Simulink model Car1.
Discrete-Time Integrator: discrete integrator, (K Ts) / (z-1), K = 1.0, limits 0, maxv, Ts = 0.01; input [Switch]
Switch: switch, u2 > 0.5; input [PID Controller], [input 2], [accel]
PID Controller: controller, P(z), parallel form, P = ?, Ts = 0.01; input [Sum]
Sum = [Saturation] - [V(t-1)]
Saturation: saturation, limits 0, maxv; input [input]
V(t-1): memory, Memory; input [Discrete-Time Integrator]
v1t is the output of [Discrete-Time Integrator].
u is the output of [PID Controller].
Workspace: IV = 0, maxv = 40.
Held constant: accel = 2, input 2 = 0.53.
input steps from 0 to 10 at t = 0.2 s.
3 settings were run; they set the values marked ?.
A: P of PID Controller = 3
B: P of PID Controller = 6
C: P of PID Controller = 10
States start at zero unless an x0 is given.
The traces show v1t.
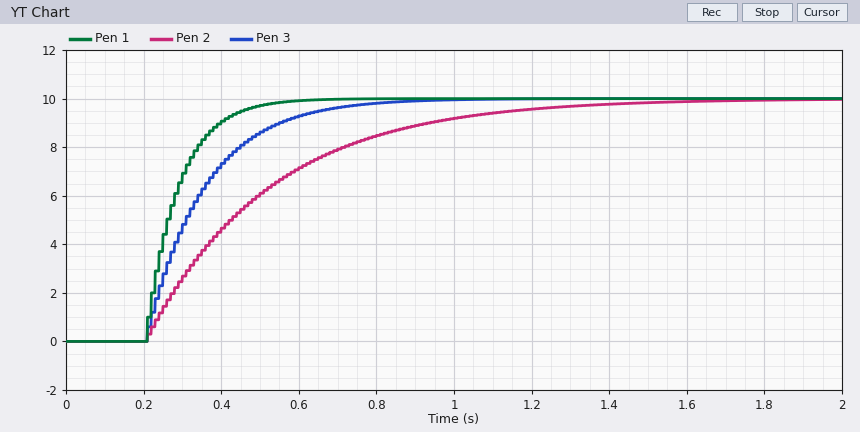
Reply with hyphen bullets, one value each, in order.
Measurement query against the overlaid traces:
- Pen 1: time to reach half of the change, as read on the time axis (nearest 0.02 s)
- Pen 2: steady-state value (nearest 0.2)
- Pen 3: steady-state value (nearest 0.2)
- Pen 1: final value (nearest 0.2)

- 0.26 s
- 10.0
- 10.0
- 10.0
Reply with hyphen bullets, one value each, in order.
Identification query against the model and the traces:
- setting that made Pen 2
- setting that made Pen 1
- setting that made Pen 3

- A
- C
- B
